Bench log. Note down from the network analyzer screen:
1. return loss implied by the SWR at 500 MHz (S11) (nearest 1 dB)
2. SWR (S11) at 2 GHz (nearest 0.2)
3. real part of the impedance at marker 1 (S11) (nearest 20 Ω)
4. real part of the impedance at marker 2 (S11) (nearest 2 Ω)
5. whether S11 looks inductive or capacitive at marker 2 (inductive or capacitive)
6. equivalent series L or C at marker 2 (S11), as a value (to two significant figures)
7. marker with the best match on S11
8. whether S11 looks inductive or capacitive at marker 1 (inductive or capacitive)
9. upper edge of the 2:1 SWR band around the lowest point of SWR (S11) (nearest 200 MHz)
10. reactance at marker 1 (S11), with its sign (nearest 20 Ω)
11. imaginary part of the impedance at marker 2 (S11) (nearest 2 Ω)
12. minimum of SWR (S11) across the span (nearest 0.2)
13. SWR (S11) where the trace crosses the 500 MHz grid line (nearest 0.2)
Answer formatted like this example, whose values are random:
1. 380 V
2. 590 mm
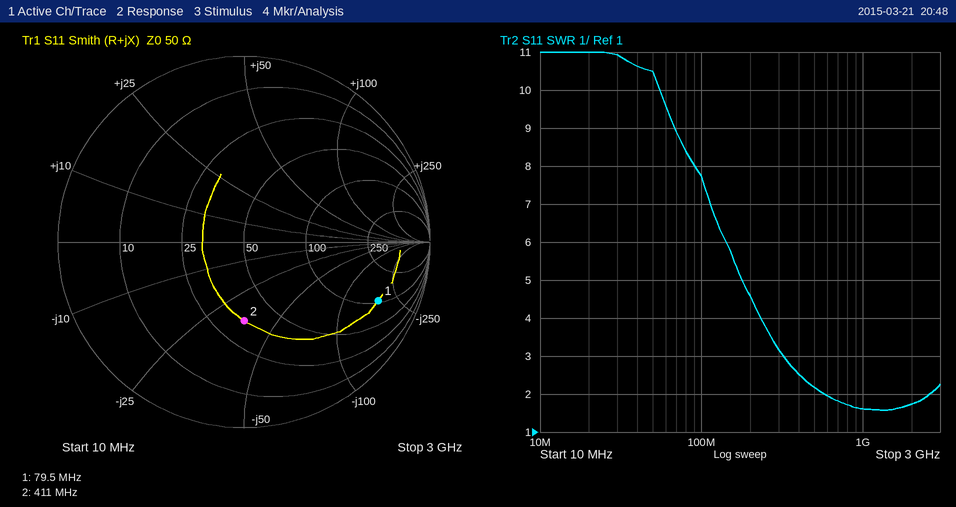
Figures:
1. 9 dB
2. 1.8
3. 100 Ω
4. 34 Ω
5. capacitive
6. 11 pF
7. marker 2
8. capacitive
9. 2.6 GHz
10. -180 Ω
11. -36 Ω
12. 1.6
13. 2.2
